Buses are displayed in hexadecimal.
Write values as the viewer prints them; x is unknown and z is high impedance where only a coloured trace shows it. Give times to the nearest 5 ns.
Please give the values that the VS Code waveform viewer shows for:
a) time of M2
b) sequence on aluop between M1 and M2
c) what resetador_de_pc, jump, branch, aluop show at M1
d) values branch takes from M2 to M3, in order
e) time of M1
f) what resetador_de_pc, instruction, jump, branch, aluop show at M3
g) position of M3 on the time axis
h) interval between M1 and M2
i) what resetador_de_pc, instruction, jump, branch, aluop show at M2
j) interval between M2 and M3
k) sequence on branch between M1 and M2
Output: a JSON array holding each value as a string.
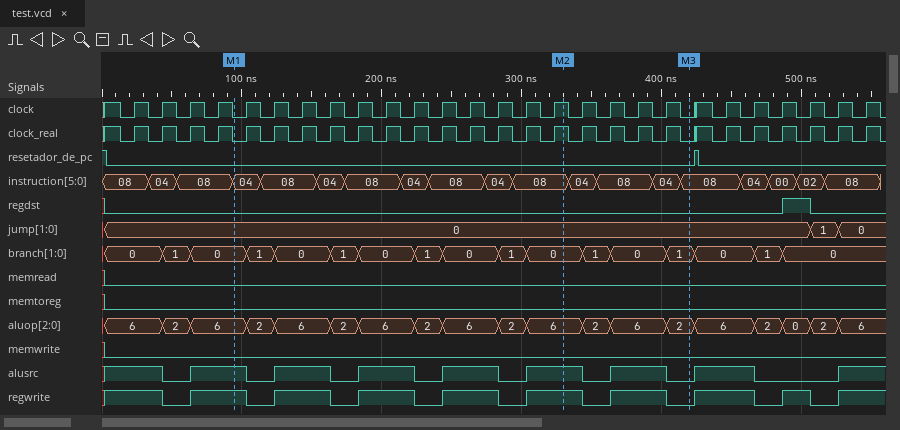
["330 ns", "6, 2, 6, 2, 6, 2, 6, 2, 6", "resetador_de_pc=0, jump=0, branch=0, aluop=6", "0, 1, 0, 1", "95 ns", "resetador_de_pc=0, instruction=08, jump=0, branch=1, aluop=2", "420 ns", "235 ns", "resetador_de_pc=0, instruction=08, jump=0, branch=0, aluop=6", "90 ns", "0, 1, 0, 1, 0, 1, 0, 1, 0"]
